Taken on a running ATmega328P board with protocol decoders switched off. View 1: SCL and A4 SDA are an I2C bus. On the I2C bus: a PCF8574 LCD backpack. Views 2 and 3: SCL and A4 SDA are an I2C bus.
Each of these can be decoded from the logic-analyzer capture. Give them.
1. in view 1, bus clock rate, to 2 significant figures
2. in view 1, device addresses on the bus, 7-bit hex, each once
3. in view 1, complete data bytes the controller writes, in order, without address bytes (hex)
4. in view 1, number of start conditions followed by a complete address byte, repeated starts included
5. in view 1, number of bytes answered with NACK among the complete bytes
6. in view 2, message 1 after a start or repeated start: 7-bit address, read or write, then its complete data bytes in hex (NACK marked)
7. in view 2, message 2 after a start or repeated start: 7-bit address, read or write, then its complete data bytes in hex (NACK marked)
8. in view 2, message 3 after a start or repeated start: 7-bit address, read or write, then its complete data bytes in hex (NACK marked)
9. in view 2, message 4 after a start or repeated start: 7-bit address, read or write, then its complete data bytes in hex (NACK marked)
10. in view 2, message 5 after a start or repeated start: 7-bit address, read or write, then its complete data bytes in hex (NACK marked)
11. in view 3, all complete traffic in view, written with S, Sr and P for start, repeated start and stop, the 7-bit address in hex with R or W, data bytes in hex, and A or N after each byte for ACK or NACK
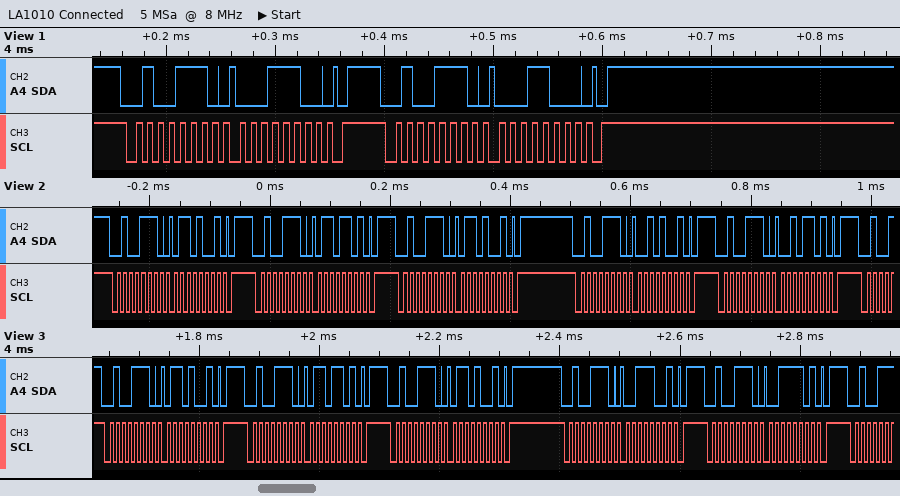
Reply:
100 kHz
0x27
1C 18
2
0
0x27 write: 69
0x27 write: 6D
0x27 write: 69
0x27 write: 29
0x27 write: 2D
S 27W A 69 A P S 27W A 6D A P S 27W A 69 A P S 27W A 39 A P S 27W A 3D A P
